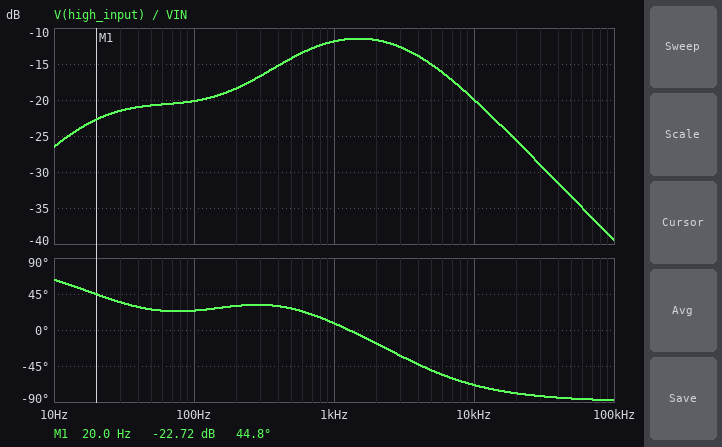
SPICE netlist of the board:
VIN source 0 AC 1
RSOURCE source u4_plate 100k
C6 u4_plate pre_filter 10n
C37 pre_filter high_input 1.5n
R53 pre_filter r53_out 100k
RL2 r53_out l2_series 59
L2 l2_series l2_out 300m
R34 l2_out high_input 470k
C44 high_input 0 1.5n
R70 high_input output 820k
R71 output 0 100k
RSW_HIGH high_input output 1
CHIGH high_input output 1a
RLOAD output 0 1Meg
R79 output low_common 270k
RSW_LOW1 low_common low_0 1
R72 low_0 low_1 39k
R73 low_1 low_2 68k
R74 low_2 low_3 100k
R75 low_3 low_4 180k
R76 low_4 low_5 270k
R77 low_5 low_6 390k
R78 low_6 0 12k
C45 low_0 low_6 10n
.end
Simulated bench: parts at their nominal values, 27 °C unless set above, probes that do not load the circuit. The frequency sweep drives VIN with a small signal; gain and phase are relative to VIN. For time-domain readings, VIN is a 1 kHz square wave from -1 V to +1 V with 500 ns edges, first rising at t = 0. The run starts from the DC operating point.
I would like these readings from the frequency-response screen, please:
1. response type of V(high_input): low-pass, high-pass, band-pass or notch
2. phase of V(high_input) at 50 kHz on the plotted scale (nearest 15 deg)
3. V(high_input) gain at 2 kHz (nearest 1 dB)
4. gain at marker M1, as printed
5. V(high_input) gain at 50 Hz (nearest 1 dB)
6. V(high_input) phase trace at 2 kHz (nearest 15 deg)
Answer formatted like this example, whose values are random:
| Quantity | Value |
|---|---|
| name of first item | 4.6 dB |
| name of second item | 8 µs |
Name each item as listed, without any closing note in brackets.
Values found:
| Quantity | Value |
|---|---|
| response type of V(high_input): low-pass, high-pass, band-pass or notch | band-pass |
| phase of V(high_input) at 50 kHz on the plotted scale | -90 deg |
| V(high_input) gain at 2 kHz | -12 dB |
| gain at marker M1, as printed | -22.72 dB |
| V(high_input) gain at 50 Hz | -21 dB |
| V(high_input) phase trace at 2 kHz | -15 deg |
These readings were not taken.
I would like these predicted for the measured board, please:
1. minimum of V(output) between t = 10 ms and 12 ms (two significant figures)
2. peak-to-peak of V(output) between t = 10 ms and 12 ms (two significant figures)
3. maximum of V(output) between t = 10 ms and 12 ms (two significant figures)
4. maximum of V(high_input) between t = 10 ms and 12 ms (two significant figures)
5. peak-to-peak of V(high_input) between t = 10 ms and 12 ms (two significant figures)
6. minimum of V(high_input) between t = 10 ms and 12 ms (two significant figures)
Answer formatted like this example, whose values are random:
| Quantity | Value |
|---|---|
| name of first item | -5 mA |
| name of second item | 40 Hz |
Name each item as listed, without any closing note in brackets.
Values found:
| Quantity | Value |
|---|---|
| minimum of V(output) between t = 10 ms and 12 ms | -320 mV |
| peak-to-peak of V(output) between t = 10 ms and 12 ms | 690 mV |
| maximum of V(output) between t = 10 ms and 12 ms | 370 mV |
| maximum of V(high_input) between t = 10 ms and 12 ms | 370 mV |
| peak-to-peak of V(high_input) between t = 10 ms and 12 ms | 690 mV |
| minimum of V(high_input) between t = 10 ms and 12 ms | -320 mV |
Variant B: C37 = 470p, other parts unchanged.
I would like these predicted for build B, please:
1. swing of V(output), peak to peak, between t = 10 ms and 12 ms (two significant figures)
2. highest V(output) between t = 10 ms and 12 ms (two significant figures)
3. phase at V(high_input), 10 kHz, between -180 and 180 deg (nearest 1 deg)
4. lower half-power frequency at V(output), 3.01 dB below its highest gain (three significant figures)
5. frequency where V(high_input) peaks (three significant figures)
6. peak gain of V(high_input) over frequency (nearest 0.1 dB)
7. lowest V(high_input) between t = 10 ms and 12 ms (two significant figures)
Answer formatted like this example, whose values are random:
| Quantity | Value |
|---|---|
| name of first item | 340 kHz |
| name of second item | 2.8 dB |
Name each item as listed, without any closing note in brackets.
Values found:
| Quantity | Value |
|---|---|
| swing of V(output), peak to peak, between t = 10 ms and 12 ms | 410 mV |
| highest V(output) between t = 10 ms and 12 ms | 230 mV |
| phase at V(high_input), 10 kHz, between -180 and 180 deg | -57 deg |
| lower half-power frequency at V(output), 3.01 dB below its highest gain | 590 Hz |
| frequency where V(high_input) peaks | 2.42 kHz |
| peak gain of V(high_input) over frequency | -15.8 dB |
| lowest V(high_input) between t = 10 ms and 12 ms | -180 mV |
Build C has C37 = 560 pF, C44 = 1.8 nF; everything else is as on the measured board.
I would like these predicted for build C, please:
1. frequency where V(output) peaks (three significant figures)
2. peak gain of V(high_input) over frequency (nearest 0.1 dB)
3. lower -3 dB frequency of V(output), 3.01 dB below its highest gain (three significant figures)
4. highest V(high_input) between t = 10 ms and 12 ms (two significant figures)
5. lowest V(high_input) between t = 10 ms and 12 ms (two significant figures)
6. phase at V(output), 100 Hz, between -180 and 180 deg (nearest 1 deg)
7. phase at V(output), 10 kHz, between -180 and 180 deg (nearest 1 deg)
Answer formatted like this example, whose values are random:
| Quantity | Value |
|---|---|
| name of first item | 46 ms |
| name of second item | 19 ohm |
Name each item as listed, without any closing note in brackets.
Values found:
| Quantity | Value |
|---|---|
| frequency where V(output) peaks | 2.03 kHz |
| peak gain of V(high_input) over frequency | -15.9 dB |
| lower -3 dB frequency of V(output), 3.01 dB below its highest gain | 493 Hz |
| highest V(high_input) between t = 10 ms and 12 ms | 230 mV |
| lowest V(high_input) between t = 10 ms and 12 ms | -170 mV |
| phase at V(output), 100 Hz, between -180 and 180 deg | 11 deg |
| phase at V(output), 10 kHz, between -180 and 180 deg | -62 deg |
